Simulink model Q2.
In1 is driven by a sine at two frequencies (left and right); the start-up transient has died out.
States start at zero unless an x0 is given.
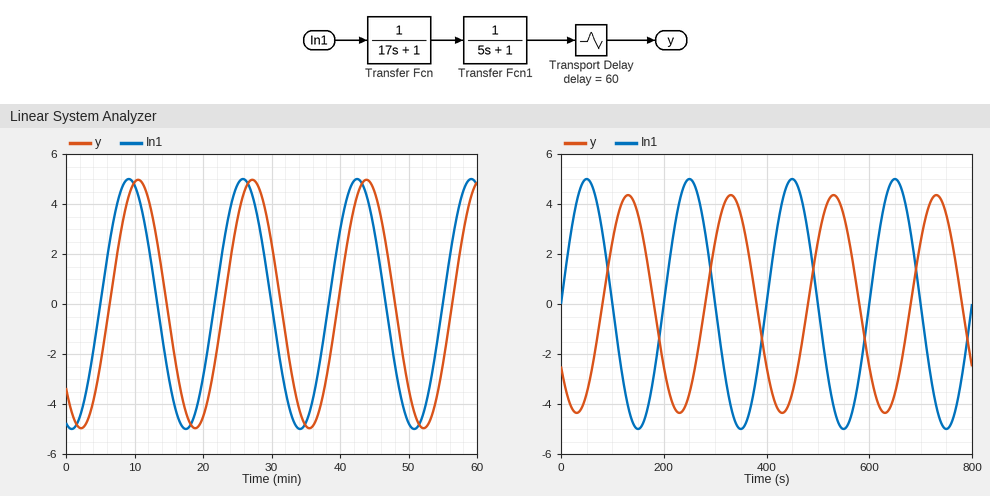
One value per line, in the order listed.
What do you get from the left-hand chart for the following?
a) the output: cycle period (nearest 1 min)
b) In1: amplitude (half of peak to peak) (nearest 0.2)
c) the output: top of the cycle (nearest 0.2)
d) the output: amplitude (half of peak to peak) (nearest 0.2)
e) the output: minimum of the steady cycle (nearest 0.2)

17 min
5.0
5.0
5.0
-5.0
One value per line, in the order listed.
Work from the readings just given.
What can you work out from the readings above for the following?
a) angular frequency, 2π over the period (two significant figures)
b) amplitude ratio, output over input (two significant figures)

0.37 rad/min
1.0
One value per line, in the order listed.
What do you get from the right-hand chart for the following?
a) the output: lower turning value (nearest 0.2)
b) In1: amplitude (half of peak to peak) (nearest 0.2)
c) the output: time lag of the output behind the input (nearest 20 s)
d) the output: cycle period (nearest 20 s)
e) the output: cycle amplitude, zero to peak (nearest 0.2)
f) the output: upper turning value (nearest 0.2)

-4.4
5.0
80 s
200 s
4.4
4.4
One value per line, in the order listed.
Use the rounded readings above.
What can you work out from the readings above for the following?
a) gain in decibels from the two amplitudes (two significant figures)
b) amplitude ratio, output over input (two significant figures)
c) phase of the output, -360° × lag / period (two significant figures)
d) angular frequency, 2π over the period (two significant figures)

-1.1 dB
0.88
-140°
0.031 rad/s
